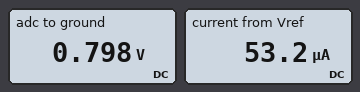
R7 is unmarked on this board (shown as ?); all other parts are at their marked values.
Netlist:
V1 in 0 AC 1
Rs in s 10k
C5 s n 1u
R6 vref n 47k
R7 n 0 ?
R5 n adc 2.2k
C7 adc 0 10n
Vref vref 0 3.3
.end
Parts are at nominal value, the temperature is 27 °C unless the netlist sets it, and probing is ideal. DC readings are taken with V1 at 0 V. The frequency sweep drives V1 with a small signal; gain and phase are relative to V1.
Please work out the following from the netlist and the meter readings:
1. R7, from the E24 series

15 kΩ
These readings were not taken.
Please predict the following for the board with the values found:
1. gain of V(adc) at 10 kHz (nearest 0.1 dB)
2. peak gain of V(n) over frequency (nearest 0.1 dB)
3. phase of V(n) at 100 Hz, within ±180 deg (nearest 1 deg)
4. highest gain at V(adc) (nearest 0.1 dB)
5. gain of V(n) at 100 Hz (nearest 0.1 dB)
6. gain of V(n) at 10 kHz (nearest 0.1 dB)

-19.2 dB
-5.5 dB
2 deg
-5.5 dB
-5.5 dB
-14.5 dB
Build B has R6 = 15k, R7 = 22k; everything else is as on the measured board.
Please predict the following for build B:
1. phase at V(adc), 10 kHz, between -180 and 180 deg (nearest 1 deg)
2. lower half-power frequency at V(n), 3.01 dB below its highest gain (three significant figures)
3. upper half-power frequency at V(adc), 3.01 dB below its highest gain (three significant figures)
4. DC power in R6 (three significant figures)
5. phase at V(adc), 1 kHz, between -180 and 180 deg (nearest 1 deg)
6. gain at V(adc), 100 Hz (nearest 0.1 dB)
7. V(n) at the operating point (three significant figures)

-77 deg
8.34 Hz
2.32 kHz
119 µW
-23 deg
-6.6 dB
1.96 V
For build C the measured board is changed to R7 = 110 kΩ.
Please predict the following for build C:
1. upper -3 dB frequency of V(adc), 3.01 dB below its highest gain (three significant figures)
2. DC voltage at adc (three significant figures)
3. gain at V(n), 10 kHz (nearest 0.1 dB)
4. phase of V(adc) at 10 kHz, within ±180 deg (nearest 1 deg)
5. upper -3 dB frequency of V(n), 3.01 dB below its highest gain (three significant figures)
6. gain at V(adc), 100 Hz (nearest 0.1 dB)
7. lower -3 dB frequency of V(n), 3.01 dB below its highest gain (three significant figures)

1.63 kHz
2.31 V
-13.6 dB
-81 deg
1.72 kHz
-2.4 dB
3.67 Hz
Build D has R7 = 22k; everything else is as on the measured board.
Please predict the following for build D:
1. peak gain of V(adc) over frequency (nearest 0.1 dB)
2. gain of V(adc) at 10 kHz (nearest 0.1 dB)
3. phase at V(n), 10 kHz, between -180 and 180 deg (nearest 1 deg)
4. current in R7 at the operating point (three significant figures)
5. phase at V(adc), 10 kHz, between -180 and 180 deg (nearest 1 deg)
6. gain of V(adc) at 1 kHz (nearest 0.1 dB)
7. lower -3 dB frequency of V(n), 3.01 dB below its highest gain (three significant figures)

-4.5 dB
-18.8 dB
-25 deg
47.8 µA
-79 deg
-5.5 dB
6.31 Hz
